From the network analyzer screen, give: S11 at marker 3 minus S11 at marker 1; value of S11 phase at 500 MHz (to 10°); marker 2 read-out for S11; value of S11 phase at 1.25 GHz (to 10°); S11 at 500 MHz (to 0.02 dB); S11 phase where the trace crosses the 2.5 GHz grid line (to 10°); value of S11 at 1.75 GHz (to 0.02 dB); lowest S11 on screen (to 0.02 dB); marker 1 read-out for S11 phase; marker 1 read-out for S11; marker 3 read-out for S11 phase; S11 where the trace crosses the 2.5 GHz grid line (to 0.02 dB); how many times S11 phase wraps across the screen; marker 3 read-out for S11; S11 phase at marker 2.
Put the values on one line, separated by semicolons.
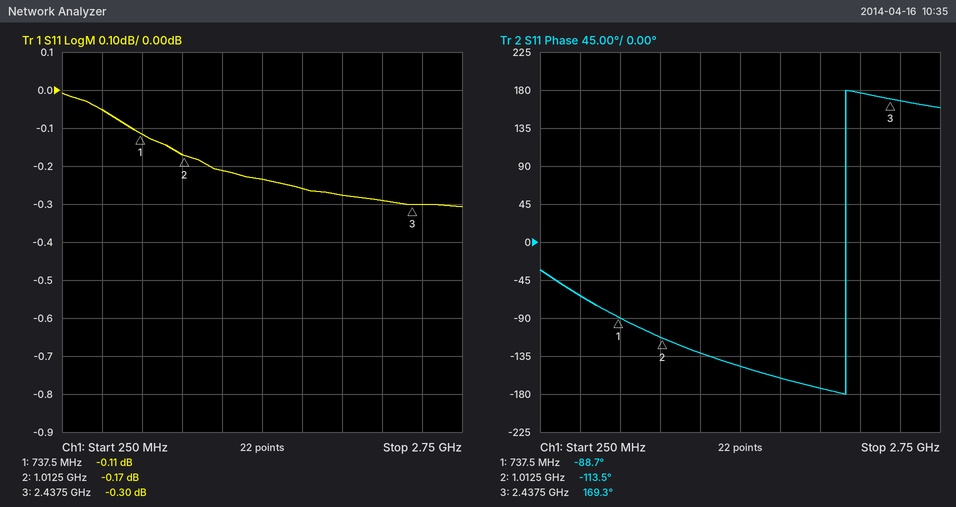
-0.19 dB; -60°; -0.17 dB; -130°; -0.06 dB; 170°; -0.26 dB; -0.30 dB; -88.7°; -0.11 dB; 169.3°; -0.30 dB; 1; -0.30 dB; -113.5°
